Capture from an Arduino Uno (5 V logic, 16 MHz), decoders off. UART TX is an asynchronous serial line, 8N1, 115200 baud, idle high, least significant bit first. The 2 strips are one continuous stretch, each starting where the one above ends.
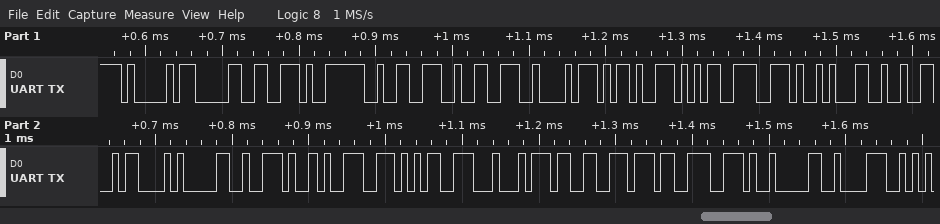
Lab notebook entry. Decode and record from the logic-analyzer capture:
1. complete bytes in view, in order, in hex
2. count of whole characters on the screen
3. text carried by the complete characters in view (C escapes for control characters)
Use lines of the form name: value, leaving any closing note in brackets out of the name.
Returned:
complete bytes in view, in order, in hex: 41 30 2E 32 32 42 2D 35 2E 31 32 43 30 2E 39 35 44 33 37 2E 30 38
count of whole characters on the screen: 22
text carried by the complete characters in view: "A0.22B-5.12C0.95D37.08"
